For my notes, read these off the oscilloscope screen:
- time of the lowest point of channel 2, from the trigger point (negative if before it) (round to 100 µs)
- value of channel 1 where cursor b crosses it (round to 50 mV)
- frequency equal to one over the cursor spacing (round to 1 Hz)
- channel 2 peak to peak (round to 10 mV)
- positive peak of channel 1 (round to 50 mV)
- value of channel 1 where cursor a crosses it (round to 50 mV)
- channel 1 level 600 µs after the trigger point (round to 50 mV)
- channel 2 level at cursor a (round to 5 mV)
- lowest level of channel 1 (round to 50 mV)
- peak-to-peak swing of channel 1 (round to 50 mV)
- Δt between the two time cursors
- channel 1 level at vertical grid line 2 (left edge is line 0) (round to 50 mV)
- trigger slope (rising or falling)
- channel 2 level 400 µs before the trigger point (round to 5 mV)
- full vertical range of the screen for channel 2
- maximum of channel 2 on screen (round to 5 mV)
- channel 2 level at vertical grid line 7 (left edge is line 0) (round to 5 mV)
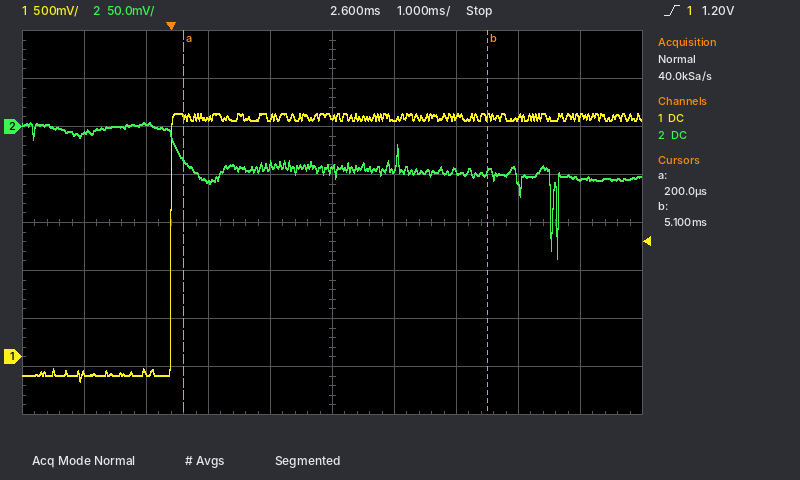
+6.2 ms
2.50 V
204 Hz
140 mV
2.55 V
2.50 V
2.50 V
-35 mV
-250 mV
2.80 V
4.9 ms
-150 mV
rising
5 mV
400 mV
5 mV
-45 mV
